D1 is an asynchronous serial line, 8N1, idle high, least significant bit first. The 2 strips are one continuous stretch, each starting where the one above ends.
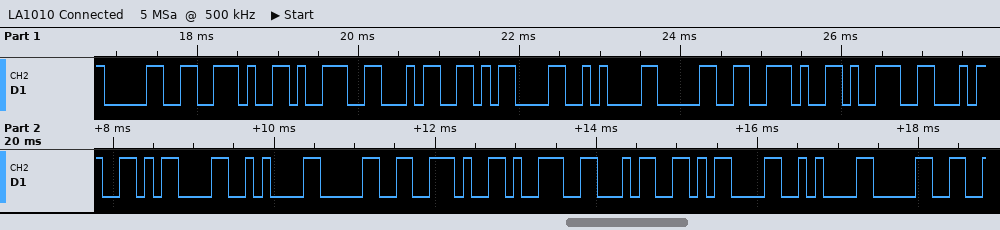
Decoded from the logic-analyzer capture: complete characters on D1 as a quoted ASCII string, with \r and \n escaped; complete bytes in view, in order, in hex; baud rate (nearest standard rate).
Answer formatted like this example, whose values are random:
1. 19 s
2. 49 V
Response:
1. "0.94\r\n0.94\r\n0.94\r\n0"
2. 30 2E 39 34 0D 0A 30 2E 39 34 0D 0A 30 2E 39 34 0D 0A 30
3. 9600 baud
